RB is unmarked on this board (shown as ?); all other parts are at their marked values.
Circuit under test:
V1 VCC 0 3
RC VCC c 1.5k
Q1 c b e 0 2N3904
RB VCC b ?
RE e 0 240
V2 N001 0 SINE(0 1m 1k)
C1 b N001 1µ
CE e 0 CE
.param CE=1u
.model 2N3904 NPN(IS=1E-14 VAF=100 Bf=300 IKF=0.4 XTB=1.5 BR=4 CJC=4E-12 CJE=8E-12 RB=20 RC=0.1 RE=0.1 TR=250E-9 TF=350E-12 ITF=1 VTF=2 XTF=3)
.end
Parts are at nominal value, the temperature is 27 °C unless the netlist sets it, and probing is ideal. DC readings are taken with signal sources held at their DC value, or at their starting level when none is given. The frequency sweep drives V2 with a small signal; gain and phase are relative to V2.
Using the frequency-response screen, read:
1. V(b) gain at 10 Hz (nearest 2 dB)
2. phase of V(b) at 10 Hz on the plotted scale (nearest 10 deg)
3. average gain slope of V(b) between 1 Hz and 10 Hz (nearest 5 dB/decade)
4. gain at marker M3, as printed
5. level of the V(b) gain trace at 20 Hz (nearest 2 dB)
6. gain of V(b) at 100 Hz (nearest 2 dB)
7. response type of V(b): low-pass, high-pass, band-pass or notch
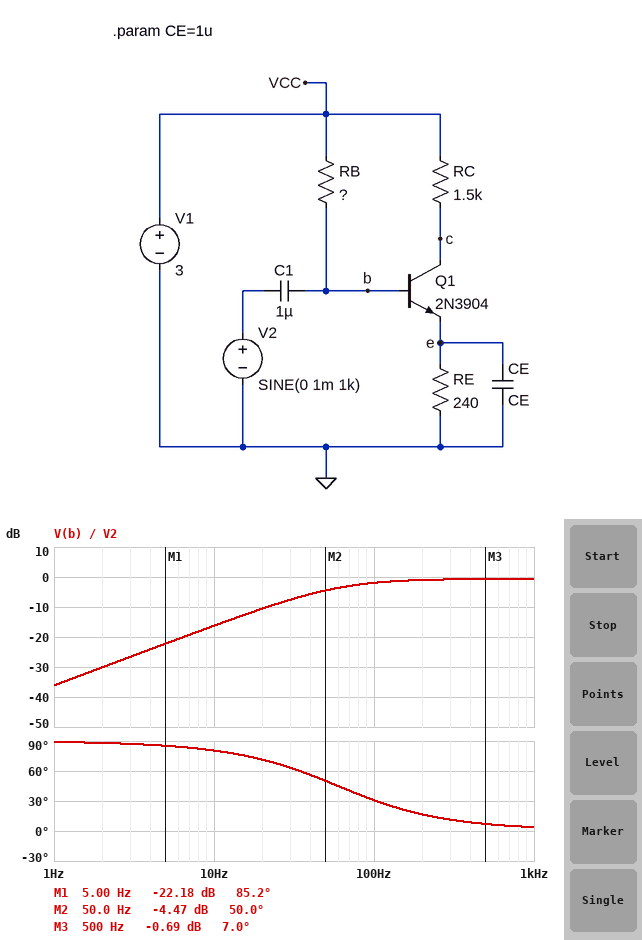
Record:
-16 dB
80 deg
20 dB/decade
-0.69 dB
-10 dB
-2 dB
high-pass
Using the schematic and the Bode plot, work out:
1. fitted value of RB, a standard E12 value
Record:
270 kΩ
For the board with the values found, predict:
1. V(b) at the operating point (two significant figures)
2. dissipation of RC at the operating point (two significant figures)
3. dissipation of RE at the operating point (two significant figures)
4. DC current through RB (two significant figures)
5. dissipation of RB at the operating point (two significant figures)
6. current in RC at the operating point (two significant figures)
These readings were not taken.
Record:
1.1 V
4.0 mW
650 µW
7.2 µA
14 µW
1.6 mA
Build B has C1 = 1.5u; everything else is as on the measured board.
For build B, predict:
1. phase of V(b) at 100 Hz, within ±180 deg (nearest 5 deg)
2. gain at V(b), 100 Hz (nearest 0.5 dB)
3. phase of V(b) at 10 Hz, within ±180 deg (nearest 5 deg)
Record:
20 deg
-1.0 dB
75 deg
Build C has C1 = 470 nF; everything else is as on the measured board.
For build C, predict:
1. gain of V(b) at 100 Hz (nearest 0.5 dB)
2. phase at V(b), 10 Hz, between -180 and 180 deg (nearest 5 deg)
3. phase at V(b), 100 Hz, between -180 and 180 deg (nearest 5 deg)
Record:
-5.0 dB
85 deg
50 deg
